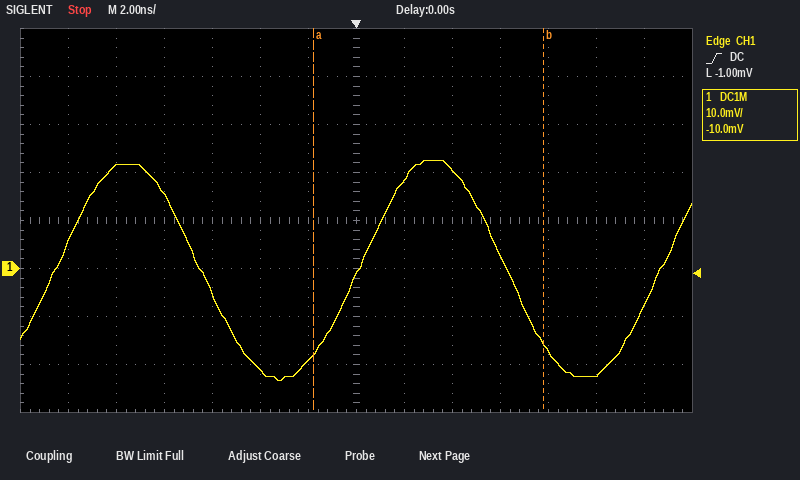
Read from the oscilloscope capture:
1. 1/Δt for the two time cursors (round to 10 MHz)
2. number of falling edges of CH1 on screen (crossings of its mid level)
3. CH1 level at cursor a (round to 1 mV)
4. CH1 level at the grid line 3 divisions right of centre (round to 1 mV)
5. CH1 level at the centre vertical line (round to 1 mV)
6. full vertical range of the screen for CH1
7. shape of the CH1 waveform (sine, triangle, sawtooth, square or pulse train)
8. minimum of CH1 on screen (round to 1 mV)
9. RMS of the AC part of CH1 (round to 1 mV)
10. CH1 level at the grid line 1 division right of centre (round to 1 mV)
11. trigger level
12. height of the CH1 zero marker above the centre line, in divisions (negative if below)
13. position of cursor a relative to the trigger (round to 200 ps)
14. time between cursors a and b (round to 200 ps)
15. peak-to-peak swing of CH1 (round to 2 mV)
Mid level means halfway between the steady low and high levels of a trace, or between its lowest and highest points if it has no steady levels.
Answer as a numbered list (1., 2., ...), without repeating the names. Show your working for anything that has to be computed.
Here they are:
1. 1 / 9.6 ns ≈ 100 MHz
2. 2
3. -18 mV
4. 3 mV
5. -1 mV
6. 80 mV
7. sine
8. -23 mV
9. 46 mV / (2√2) ≈ 16 mV
10. 18 mV
11. -1.00 mV
12. -1.0 div
13. -1.8 ns
14. 9.6 ns
15. 46 mV
